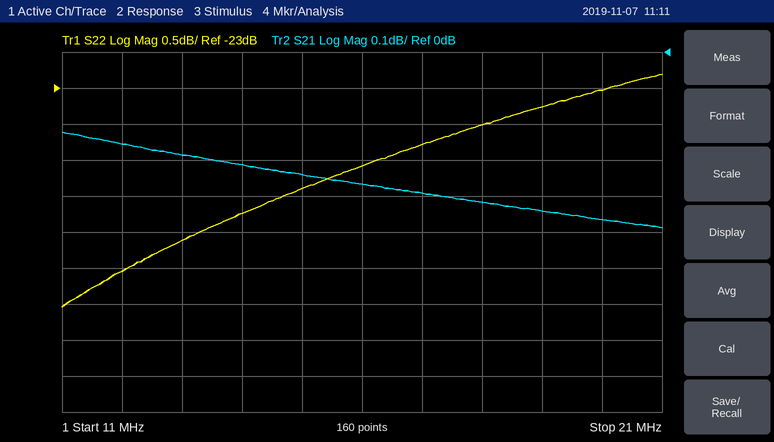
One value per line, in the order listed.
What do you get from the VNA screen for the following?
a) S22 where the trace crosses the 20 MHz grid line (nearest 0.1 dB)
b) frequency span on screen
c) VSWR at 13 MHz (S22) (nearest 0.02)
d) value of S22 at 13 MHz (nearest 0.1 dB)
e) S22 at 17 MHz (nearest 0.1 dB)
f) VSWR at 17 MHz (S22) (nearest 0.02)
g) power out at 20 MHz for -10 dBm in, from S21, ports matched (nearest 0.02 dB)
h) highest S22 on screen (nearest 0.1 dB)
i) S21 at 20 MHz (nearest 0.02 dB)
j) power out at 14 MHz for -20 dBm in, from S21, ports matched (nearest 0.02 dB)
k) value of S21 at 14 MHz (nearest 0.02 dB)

-23.0 dB
10 MHz
1.12
-25.1 dB
-23.8 dB
1.14
-10.46 dBm
-22.8 dB
-0.46 dB
-20.32 dBm
-0.32 dB
